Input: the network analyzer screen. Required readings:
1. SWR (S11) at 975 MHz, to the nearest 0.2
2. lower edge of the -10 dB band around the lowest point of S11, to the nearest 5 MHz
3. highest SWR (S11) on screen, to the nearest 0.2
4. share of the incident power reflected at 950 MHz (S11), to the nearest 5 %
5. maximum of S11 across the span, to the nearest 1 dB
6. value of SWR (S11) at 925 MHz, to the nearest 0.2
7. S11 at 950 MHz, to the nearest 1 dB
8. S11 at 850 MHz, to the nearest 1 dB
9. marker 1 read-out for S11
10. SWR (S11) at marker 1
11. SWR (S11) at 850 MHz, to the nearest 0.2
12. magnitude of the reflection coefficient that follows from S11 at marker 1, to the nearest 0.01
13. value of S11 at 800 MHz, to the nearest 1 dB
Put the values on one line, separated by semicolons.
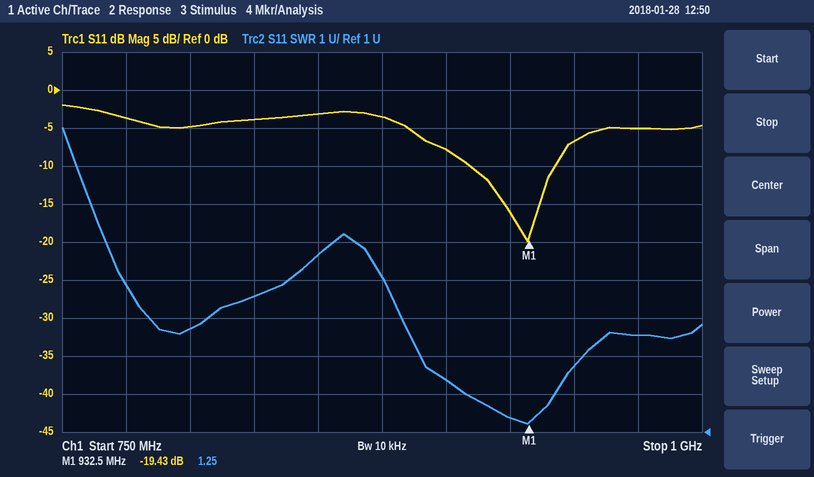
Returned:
3.6; 910 MHz; 9.0; 20 %; -2 dB; 1.4; -7 dB; -3 dB; -19.43 dB; 1.25; 5.6; 0.11; -5 dB
